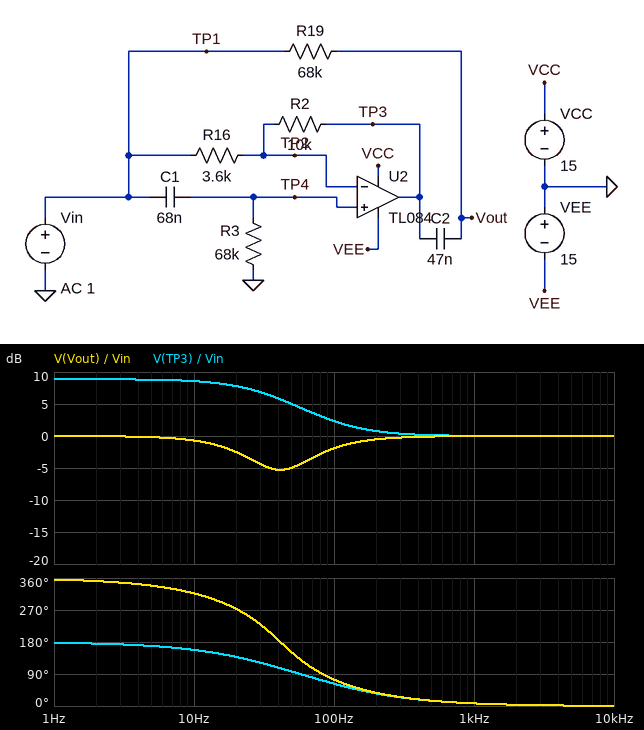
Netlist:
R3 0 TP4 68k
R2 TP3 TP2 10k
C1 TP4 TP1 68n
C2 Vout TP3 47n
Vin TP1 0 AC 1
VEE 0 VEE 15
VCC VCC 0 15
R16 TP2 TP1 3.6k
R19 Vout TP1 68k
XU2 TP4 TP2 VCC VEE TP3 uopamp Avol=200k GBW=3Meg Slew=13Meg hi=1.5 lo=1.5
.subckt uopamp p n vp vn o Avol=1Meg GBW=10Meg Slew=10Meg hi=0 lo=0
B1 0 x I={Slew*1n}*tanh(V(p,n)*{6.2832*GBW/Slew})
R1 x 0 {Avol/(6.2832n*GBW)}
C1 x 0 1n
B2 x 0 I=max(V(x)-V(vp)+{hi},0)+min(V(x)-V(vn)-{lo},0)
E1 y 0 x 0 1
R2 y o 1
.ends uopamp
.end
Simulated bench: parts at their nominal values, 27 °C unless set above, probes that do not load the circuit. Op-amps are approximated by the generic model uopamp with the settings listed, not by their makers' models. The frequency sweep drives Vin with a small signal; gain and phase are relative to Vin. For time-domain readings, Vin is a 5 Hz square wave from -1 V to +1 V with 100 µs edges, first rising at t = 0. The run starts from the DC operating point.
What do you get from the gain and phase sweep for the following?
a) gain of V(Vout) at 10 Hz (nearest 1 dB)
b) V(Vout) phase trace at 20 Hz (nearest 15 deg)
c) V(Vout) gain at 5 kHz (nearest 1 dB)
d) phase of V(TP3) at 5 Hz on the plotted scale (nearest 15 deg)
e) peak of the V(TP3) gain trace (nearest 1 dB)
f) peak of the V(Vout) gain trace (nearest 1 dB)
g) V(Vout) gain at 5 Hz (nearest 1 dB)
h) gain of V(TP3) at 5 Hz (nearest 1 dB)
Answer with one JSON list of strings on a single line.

["-1 dB", "270 deg", "0 dB", "165 deg", "9 dB", "0 dB", "0 dB", "9 dB"]
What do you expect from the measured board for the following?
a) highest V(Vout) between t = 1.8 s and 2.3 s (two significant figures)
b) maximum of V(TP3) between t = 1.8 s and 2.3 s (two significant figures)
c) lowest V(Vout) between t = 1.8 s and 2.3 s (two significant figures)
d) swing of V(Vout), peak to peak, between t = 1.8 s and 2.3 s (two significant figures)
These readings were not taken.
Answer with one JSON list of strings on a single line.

["1.3 V", "4.7 V", "-1.3 V", "2.6 V"]
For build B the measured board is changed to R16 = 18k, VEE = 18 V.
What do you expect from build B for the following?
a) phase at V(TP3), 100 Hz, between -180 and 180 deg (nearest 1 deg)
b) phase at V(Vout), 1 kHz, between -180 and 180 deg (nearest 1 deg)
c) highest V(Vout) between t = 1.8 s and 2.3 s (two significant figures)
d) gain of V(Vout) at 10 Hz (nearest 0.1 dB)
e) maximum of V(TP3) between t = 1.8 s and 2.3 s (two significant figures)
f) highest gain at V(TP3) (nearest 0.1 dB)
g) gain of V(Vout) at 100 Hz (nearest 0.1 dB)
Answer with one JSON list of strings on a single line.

["30 deg", "3 deg", "1.0 V", "-0.9 dB", "2.5 V", "0 dB", "-2.5 dB"]
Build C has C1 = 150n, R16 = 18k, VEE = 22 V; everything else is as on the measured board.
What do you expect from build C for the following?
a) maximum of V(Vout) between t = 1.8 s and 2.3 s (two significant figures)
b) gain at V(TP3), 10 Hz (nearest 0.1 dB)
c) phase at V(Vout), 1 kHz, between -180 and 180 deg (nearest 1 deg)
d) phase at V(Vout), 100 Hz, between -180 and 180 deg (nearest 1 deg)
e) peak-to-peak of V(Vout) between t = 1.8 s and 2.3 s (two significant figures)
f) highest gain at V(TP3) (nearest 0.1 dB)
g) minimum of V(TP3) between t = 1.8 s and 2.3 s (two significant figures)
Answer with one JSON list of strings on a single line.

["1.0 V", "-2.9 dB", "1 deg", "11 deg", "2.0 V", "0 dB", "-2.5 V"]
